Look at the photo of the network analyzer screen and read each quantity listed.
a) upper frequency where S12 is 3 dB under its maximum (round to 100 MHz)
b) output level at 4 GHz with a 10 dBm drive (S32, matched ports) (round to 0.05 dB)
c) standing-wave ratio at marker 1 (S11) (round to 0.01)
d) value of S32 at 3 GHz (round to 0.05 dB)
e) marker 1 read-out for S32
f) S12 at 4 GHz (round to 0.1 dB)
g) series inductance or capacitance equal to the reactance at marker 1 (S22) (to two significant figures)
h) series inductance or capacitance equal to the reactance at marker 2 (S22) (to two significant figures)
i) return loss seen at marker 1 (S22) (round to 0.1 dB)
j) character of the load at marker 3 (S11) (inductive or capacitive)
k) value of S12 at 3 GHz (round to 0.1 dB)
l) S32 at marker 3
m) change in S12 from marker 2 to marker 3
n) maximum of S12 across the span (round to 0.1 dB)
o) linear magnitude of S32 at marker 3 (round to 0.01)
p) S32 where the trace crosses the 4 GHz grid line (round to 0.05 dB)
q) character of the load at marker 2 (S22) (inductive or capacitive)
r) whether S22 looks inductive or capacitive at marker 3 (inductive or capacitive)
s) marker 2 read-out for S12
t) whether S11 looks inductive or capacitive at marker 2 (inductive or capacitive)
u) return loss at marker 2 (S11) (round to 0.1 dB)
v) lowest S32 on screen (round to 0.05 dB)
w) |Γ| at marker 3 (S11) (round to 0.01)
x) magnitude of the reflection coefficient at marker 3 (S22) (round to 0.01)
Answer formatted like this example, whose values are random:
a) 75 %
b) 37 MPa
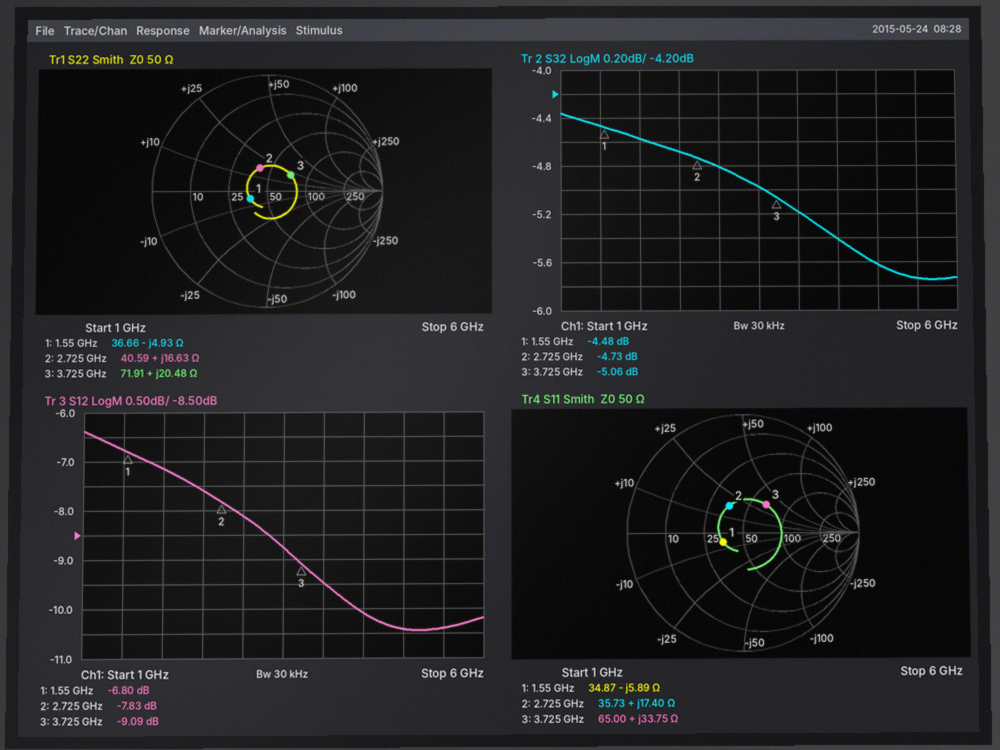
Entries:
a) 3.9 GHz
b) 4.80 dBm
c) 1.47
d) -4.80 dB
e) -4.48 dB
f) -9.5 dB
g) 21 pF
h) 970 pH
i) 15.7 dB
j) inductive
k) -8.1 dB
l) -5.06 dB
m) -1.26 dB
n) -6.4 dB
o) 0.56
p) -5.20 dB
q) inductive
r) inductive
s) -7.83 dB
t) inductive
u) 11.8 dB
v) -5.75 dB
w) 0.31
x) 0.24
